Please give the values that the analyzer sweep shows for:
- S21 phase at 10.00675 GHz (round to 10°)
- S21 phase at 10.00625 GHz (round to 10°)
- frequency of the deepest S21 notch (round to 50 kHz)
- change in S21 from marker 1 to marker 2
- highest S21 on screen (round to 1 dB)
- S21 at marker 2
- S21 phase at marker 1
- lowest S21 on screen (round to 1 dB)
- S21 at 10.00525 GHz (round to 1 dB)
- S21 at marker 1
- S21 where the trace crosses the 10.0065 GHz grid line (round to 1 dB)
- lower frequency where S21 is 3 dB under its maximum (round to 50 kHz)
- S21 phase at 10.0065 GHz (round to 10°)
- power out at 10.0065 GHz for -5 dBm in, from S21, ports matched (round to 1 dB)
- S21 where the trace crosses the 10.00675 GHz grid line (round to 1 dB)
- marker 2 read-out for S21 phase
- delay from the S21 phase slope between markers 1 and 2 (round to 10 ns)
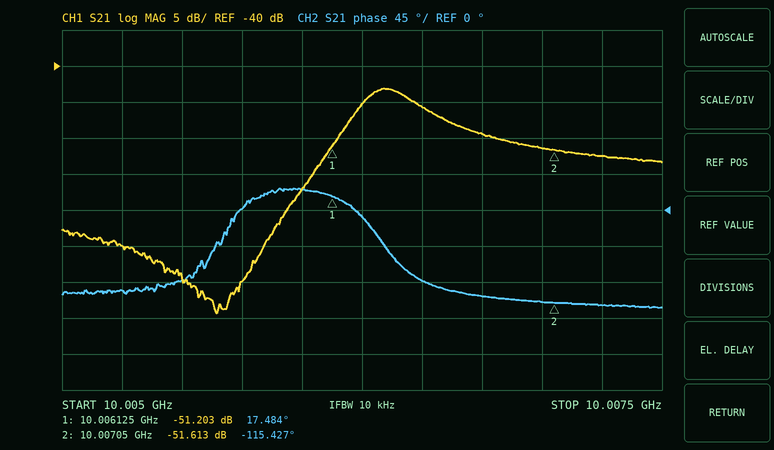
-110°
-10°
10.00565 GHz
-0.410 dB
-43 dB
-51.613 dB
17.484°
-74 dB
-65 dB
-51.203 dB
-46 dB
10.00625 GHz
-90°
-51 dBm
-49 dB
-115.427°
400 ns
